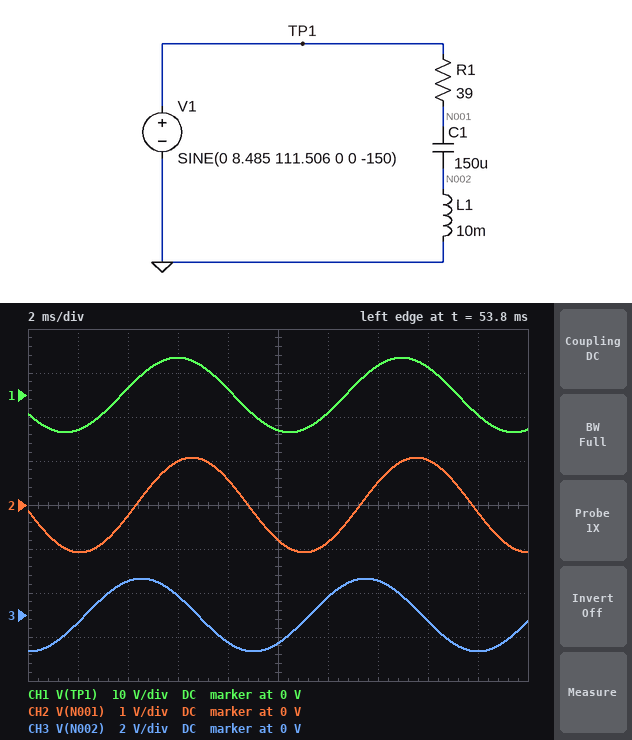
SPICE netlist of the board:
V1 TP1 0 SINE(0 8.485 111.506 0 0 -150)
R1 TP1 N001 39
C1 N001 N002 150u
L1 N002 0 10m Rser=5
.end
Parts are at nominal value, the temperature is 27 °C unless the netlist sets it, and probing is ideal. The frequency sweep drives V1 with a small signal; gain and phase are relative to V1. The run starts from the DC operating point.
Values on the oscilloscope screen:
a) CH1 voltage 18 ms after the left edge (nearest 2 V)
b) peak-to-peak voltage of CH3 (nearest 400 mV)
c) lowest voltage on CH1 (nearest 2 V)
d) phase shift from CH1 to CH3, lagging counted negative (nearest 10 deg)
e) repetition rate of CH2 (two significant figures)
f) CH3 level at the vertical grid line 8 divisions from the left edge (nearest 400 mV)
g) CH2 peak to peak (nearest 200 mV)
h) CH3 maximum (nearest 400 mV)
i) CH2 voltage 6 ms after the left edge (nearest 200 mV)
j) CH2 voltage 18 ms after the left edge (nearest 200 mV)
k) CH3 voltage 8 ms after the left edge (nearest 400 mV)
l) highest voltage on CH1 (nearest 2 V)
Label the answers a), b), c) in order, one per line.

a) -4 V
b) 3.2 V
c) -8 V
d) 60 deg
e) 110 Hz
f) -400 mV
g) 2.2 V
h) 1.6 V
i) 1.0 V
j) -200 mV
k) -1.2 V
l) 8 V
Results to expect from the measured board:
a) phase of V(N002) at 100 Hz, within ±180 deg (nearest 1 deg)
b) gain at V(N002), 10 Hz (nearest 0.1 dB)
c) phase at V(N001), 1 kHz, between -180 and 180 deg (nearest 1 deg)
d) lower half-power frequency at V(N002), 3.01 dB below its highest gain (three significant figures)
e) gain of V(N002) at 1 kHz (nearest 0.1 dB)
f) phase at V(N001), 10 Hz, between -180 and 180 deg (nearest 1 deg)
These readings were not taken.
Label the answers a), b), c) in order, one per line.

a) 57 deg
b) -27.1 dB
c) 31 deg
d) 667 Hz
e) -1.6 dB
f) -20 deg
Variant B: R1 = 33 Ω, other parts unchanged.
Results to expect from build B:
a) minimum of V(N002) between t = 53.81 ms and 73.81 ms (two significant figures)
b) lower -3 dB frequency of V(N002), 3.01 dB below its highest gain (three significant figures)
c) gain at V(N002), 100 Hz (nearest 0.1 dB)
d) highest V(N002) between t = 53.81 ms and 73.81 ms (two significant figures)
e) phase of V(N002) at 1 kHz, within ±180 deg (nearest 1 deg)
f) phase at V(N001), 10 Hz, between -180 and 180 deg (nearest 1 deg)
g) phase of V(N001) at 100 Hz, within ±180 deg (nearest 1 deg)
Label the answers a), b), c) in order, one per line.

a) -1.9 V
b) 566 Hz
c) -13.6 dB
d) 1.9 V
e) 27 deg
f) -17 deg
g) -34 deg
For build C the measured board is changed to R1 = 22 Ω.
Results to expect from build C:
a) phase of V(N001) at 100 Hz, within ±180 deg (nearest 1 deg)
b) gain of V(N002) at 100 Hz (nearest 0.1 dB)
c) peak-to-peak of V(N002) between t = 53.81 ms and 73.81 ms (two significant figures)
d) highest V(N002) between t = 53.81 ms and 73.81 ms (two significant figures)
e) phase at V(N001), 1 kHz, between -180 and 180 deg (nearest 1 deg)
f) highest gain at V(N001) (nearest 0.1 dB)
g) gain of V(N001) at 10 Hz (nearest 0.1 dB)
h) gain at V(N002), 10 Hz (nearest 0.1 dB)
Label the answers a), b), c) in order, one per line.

a) -32 deg
b) -10.6 dB
c) 5.4 V
d) 2.7 V
e) 19 deg
f) 0 dB
g) -0.3 dB
h) -26.7 dB
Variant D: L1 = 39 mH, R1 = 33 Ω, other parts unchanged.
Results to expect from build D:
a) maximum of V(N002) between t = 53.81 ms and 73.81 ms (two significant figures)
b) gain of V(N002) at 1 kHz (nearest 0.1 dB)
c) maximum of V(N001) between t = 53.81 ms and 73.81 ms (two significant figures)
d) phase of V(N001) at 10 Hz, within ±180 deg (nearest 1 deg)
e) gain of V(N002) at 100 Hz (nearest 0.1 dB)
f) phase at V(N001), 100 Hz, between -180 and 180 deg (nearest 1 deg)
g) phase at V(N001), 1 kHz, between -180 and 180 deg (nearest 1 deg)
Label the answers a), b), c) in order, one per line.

a) 5.6 V
b) -0.1 dB
c) 3.7 V
d) -17 deg
e) -4.2 dB
f) 50 deg
g) 8 deg
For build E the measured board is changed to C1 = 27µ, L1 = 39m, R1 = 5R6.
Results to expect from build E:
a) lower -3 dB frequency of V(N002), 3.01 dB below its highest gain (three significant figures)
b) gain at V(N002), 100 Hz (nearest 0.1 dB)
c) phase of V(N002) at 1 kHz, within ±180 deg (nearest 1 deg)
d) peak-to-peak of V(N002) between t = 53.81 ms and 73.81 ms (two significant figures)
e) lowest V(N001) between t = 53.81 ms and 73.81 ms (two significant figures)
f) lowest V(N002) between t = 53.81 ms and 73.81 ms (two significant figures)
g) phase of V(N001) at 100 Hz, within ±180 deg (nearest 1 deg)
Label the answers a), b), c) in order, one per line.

a) 139 Hz
b) -3.2 dB
c) 1 deg
d) 17 V
e) -8.0 V
f) -8.5 V
g) -9 deg
